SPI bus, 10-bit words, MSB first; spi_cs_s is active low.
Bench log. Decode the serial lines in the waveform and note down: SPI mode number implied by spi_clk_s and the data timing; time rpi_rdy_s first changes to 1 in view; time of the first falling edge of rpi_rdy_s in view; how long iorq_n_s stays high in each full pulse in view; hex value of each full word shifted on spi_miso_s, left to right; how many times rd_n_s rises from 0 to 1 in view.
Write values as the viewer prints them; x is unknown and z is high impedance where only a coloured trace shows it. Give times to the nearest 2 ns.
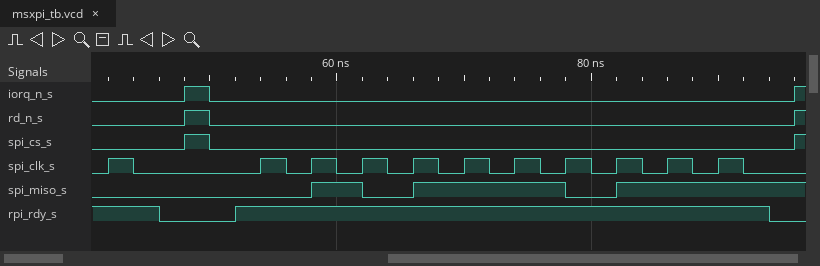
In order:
1
52 ns
46 ns
2 ns
177
2
